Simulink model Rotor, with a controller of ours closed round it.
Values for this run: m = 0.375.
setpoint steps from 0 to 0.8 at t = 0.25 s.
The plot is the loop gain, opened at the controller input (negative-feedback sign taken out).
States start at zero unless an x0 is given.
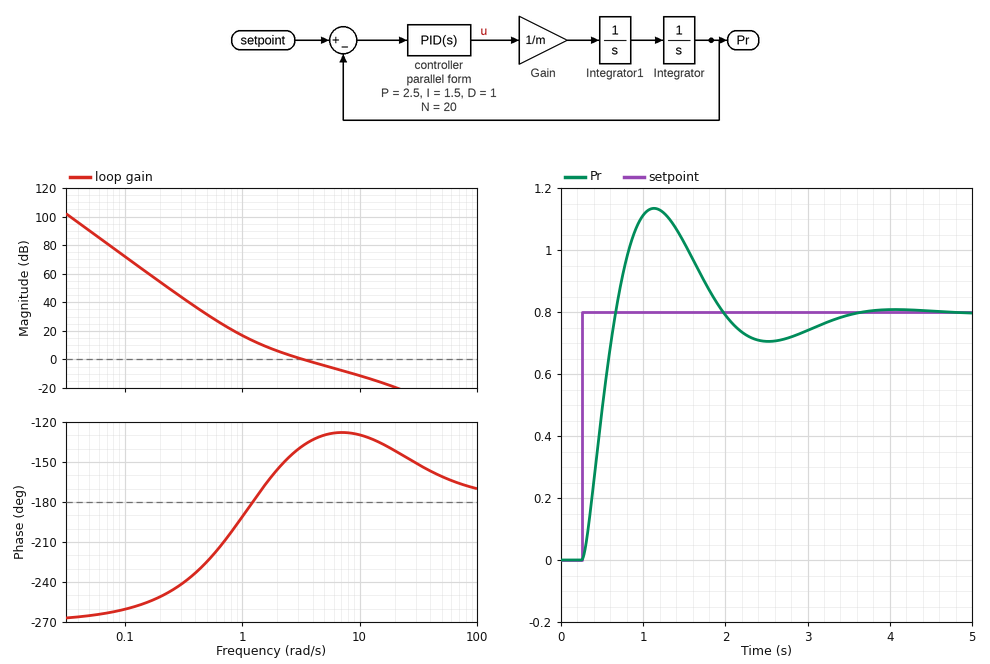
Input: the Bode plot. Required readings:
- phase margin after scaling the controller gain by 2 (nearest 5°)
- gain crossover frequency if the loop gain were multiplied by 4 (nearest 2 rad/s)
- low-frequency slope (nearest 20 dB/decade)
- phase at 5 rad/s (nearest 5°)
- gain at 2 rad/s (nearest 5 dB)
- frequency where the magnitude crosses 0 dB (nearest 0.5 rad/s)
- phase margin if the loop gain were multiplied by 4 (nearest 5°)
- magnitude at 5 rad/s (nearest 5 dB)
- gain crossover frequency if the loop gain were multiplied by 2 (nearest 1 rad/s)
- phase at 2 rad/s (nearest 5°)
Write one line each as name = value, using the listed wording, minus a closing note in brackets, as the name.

phase margin after scaling the controller gain by 2 = 50°
gain crossover frequency if the loop gain were multiplied by 4 = 10 rad/s
low-frequency slope = -60 dB/decade
phase at 5 rad/s = -130°
gain at 2 rad/s = 5 dB
frequency where the magnitude crosses 0 dB = 3.5 rad/s
phase margin if the loop gain were multiplied by 4 = 50°
magnitude at 5 rad/s = -5 dB
gain crossover frequency if the loop gain were multiplied by 2 = 6 rad/s
phase at 2 rad/s = -155°
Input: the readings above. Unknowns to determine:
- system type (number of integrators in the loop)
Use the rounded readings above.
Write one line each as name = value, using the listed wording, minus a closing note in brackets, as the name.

system type = 3
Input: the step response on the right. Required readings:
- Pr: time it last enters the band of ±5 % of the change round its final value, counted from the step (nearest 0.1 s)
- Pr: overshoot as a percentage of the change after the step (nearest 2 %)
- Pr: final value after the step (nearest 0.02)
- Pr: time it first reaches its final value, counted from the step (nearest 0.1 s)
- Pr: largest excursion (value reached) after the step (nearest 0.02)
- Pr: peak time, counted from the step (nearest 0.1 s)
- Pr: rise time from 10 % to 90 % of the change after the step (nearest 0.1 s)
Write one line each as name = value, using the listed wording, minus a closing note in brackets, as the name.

Pr: time it last enters the band of ±5 % of the change round its final value, counted from the step = 2.9 s
Pr: overshoot as a percentage of the change after the step = 42 %
Pr: final value after the step = 0.80
Pr: time it first reaches its final value, counted from the step = 0.4 s
Pr: largest excursion (value reached) after the step = 1.14
Pr: peak time, counted from the step = 0.9 s
Pr: rise time from 10 % to 90 % of the change after the step = 0.3 s
